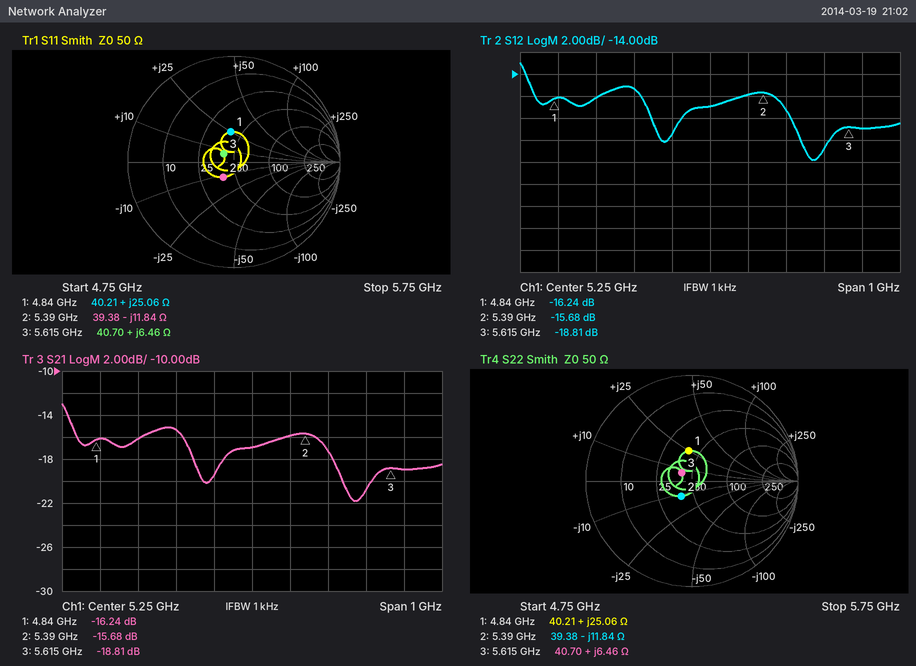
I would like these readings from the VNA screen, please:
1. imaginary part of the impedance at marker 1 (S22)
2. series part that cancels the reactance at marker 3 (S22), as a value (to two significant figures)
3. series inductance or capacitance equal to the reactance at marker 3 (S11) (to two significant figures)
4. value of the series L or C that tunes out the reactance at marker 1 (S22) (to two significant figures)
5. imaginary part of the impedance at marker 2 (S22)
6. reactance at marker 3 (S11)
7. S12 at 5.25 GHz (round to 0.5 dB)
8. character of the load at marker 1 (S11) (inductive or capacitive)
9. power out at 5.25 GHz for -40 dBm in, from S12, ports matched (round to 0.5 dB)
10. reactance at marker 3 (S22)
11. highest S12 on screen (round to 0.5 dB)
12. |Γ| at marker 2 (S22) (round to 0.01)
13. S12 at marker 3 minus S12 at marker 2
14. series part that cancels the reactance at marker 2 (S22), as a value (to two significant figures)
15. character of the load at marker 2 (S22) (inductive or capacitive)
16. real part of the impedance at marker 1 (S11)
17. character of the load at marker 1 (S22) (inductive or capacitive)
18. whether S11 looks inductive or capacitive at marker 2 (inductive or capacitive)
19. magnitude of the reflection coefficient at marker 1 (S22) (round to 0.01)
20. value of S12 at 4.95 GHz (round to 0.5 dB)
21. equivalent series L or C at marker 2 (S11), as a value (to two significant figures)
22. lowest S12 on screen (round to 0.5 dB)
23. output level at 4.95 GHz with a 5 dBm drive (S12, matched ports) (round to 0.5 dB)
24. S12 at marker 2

+25.06 Ω
4.4 pF
180 pH
1.3 pF
-11.84 Ω
+6.46 Ω
-17.0 dB
inductive
-57.0 dBm
+6.46 Ω
-13.0 dB
0.18
-3.13 dB
350 pH
capacitive
40.21 Ω
inductive
capacitive
0.29
-16.0 dB
2.5 pF
-22.0 dB
-11.0 dBm
-15.68 dB
